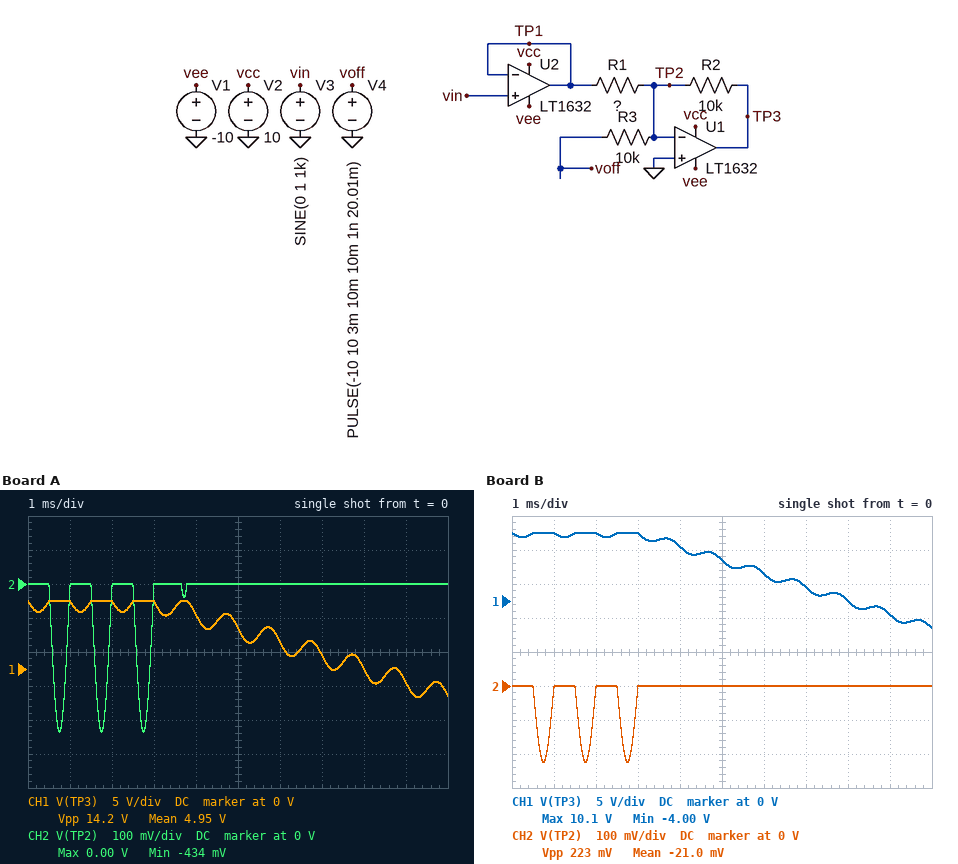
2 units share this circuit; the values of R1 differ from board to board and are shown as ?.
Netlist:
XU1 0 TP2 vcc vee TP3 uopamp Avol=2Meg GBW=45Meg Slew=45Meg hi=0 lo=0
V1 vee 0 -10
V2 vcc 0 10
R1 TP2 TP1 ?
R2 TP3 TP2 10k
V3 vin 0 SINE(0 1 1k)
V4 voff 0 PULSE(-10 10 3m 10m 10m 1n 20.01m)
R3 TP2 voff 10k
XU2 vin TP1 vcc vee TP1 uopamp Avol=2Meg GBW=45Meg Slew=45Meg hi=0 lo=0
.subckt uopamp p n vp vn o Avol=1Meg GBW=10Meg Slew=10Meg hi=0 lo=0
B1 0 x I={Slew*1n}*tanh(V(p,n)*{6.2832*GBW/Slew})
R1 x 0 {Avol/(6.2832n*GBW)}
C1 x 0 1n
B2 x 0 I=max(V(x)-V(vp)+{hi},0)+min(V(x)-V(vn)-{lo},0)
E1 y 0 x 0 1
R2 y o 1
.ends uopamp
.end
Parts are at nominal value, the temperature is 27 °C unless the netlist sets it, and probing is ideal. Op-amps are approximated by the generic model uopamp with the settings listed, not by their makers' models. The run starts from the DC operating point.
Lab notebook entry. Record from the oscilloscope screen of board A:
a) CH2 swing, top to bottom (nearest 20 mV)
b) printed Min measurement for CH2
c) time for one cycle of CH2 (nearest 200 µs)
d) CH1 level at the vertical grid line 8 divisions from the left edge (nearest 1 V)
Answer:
440 mV
-434 mV
1.0 ms
0 V
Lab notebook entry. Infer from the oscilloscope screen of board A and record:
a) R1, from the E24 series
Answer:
6.2 kΩ
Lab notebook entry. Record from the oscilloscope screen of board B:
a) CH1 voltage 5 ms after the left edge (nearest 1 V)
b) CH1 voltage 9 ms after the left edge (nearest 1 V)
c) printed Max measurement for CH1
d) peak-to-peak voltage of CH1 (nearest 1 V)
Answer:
6 V
-2 V
10.1 V
14 V
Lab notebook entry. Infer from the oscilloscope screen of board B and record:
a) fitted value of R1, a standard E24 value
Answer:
16 kΩ
